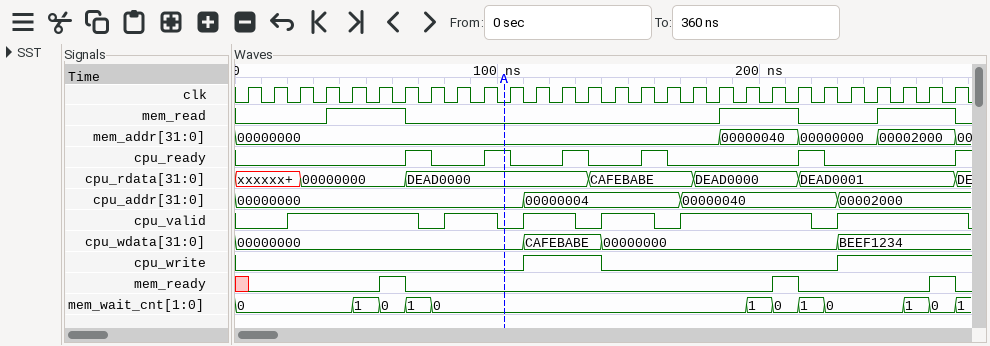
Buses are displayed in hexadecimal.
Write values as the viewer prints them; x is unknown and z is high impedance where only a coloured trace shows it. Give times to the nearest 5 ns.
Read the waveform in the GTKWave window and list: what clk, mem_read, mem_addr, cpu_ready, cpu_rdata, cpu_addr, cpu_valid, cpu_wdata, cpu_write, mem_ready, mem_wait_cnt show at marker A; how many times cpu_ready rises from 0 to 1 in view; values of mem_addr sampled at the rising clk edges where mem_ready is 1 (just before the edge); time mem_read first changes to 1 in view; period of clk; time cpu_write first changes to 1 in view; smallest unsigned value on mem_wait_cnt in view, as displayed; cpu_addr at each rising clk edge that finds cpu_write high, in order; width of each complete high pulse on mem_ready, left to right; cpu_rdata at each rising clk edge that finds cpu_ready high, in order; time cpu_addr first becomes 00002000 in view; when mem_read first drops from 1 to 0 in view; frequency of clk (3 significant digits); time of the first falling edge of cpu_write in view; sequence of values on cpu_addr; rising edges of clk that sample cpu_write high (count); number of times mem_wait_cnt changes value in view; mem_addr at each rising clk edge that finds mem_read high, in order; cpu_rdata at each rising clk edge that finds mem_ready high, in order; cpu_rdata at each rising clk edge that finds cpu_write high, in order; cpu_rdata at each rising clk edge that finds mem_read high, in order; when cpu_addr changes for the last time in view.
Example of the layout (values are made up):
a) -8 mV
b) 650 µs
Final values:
a) clk=0, mem_read=0, mem_addr=00000000, cpu_ready=1, cpu_rdata=DEAD0000, cpu_addr=00000000, cpu_valid=0, cpu_wdata=00000000, cpu_write=0, mem_ready=0, mem_wait_cnt=0
b) 6
c) 00000000, 00000040, 00002000
d) 35 ns
e) 10 ns
f) 110 ns
g) 0
h) 00000004, 00000004, 00000004, 00002000, 00002000, 00002000, 00002000, 00002000
i) 10 ns, 10 ns, 10 ns
j) DEAD0000, DEAD0000, DEAD0000, CAFEBABE, DEAD0001
k) 230 ns
l) 65 ns
m) 100 MHz
n) 140 ns
o) 00000000, 00000004, 00000040, 00002000
p) 8
q) 11
r) 00000000, 00000000, 00000000, 00000040, 00000040, 00000040, 00002000, 00002000, 00002000
s) 00000000, DEAD0000, DEAD0001
t) DEAD0000, DEAD0000, DEAD0000, DEAD0001, DEAD0001, DEAD0001, DEAD0001, DEAD0001
u) 00000000, 00000000, 00000000, DEAD0000, DEAD0000, DEAD0000, DEAD0001, DEAD0001, DEAD0001
v) 230 ns
